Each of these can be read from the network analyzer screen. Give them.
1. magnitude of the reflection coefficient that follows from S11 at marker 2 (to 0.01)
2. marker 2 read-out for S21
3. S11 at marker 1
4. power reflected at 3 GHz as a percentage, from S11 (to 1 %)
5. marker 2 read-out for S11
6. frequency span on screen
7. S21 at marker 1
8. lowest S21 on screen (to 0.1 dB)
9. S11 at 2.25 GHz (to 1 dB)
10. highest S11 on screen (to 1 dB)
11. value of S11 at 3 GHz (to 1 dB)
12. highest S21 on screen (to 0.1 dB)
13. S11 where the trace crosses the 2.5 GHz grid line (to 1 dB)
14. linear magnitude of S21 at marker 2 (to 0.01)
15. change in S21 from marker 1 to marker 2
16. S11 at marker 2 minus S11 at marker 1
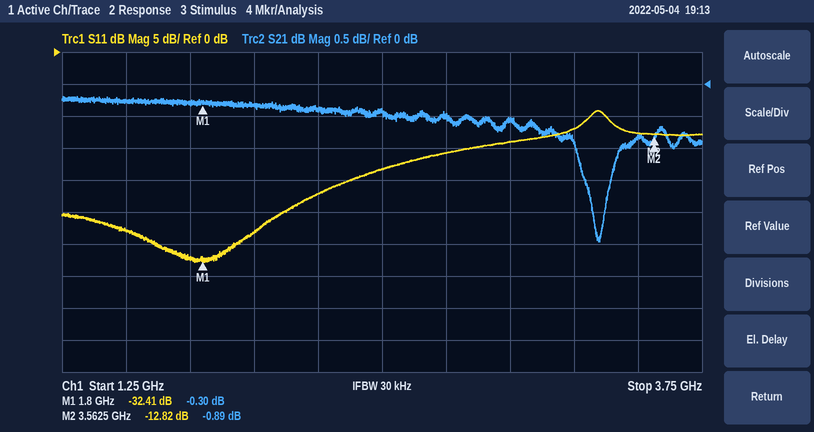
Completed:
0.23
-0.89 dB
-32.41 dB
4 %
-12.82 dB
2.5 GHz
-0.30 dB
-2.5 dB
-22 dB
-9 dB
-14 dB
-0.2 dB
-18 dB
0.90
-0.59 dB
19.59 dB
